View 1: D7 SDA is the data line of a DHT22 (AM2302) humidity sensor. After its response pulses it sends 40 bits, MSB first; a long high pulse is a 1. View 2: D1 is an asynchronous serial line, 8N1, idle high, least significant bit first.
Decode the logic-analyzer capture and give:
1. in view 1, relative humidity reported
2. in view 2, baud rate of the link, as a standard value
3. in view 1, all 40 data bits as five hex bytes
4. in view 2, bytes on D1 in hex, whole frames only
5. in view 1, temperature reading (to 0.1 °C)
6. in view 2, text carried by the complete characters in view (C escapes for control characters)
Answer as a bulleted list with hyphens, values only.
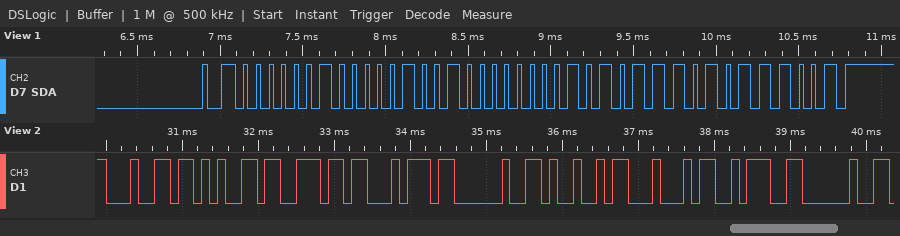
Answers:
- 52.1 %
- 9600 baud
- 02 09 00 AE B9
- 64 65 6E 74 20 49 44 3A 20
- 17.4 °C
- "dent ID: "
